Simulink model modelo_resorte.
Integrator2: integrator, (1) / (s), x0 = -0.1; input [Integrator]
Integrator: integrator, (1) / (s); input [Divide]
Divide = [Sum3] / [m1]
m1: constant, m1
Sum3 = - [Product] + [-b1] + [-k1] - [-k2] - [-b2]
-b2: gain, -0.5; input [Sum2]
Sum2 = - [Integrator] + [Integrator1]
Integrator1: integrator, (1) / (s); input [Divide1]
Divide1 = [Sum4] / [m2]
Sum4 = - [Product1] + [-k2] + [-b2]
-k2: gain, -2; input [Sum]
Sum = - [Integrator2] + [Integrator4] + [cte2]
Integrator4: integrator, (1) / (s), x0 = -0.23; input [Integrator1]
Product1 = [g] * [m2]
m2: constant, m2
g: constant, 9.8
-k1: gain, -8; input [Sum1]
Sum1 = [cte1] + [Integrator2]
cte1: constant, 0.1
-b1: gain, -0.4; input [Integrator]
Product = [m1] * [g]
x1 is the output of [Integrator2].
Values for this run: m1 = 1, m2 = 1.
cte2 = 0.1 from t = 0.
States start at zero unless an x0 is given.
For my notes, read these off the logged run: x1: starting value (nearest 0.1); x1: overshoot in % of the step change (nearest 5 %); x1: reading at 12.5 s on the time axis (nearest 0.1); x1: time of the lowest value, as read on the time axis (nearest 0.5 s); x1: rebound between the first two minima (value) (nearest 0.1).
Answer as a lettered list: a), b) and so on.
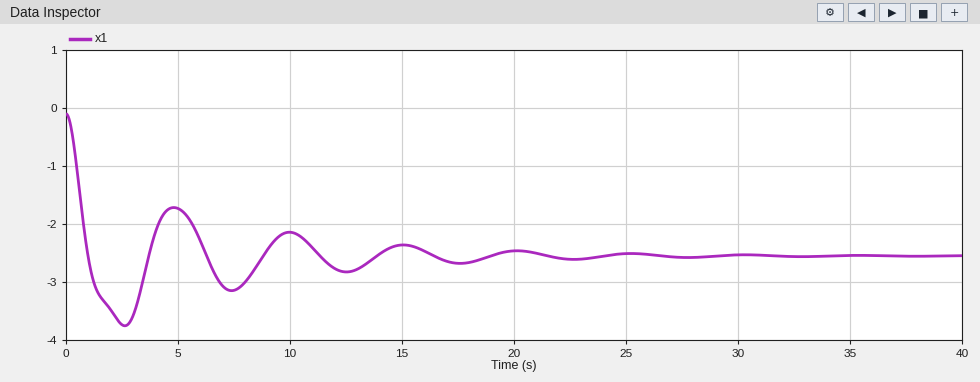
a) -0.1
b) 50 %
c) -2.8
d) 2.5 s
e) -1.7
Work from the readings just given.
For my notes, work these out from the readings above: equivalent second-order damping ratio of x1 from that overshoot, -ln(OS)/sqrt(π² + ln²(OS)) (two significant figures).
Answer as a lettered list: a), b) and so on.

a) 0.22
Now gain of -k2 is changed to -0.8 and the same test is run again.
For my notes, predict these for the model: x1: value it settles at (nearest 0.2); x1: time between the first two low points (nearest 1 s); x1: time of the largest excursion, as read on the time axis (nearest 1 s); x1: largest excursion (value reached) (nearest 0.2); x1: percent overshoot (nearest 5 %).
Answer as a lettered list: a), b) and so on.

a) -2.6
b) 7 s
c) 3 s
d) -3.6
e) 40 %
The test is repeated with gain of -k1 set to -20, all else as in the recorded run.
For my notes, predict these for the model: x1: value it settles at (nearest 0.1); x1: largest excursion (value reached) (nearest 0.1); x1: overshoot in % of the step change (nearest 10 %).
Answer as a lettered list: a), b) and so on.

a) -1.1
b) -1.6
c) 50 %
